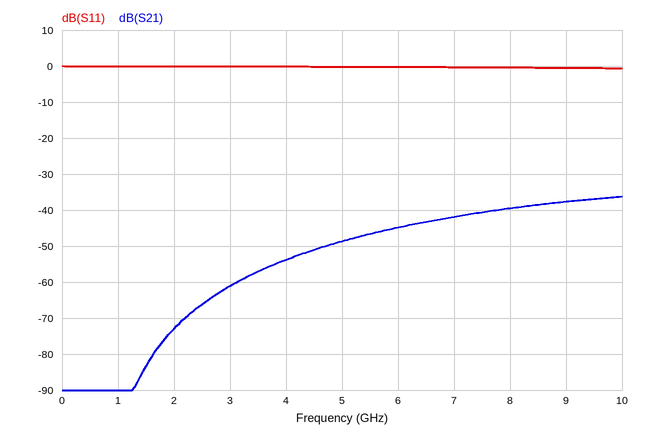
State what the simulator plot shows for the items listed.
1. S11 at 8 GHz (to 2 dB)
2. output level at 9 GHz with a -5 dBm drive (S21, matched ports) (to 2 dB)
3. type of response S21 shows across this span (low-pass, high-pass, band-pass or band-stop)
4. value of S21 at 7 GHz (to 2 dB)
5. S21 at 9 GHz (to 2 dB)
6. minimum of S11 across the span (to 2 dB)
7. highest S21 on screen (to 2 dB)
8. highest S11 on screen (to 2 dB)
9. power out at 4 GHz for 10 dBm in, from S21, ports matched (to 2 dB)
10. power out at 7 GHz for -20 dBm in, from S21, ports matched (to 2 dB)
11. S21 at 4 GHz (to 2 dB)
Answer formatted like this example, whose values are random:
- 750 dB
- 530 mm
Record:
- 0 dB
- -42 dBm
- high-pass
- -42 dB
- -38 dB
- 0 dB
- -36 dB
- 0 dB
- -44 dBm
- -62 dBm
- -54 dB
